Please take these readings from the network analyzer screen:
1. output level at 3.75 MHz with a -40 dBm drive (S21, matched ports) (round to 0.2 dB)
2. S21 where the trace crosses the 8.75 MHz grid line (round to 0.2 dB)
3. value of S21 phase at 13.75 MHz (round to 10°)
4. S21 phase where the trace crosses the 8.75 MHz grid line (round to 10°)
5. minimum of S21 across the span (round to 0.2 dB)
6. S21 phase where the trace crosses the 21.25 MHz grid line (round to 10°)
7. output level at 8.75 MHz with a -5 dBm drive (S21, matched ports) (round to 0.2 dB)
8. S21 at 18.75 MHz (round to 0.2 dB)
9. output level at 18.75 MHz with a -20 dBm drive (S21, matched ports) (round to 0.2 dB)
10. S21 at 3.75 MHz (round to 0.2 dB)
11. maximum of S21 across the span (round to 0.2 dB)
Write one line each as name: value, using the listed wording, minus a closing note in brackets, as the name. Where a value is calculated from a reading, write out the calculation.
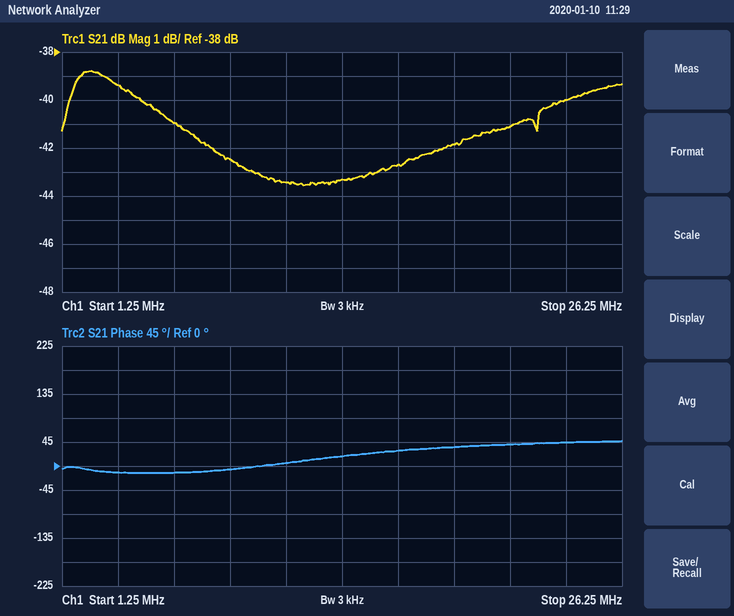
output level at 3.75 MHz with a -40 dBm drive (S21, matched ports): -40 dBm + (-39.4 dB) = -79.4 dBm
S21 where the trace crosses the 8.75 MHz grid line: -42.4 dB
value of S21 phase at 13.75 MHz: 20°
S21 phase where the trace crosses the 8.75 MHz grid line: -10°
minimum of S21 across the span: -43.6 dB
S21 phase where the trace crosses the 21.25 MHz grid line: 40°
output level at 8.75 MHz with a -5 dBm drive (S21, matched ports): -5 dBm + (-42.4 dB) = -47.4 dBm
S21 at 18.75 MHz: -41.8 dB
output level at 18.75 MHz with a -20 dBm drive (S21, matched ports): -20 dBm + (-41.8 dB) = -61.8 dBm
S21 at 3.75 MHz: -39.4 dB
maximum of S21 across the span: -38.8 dB
